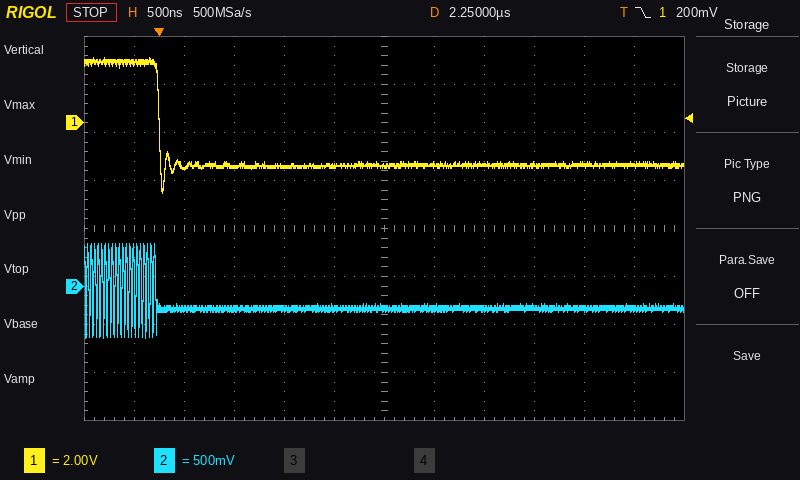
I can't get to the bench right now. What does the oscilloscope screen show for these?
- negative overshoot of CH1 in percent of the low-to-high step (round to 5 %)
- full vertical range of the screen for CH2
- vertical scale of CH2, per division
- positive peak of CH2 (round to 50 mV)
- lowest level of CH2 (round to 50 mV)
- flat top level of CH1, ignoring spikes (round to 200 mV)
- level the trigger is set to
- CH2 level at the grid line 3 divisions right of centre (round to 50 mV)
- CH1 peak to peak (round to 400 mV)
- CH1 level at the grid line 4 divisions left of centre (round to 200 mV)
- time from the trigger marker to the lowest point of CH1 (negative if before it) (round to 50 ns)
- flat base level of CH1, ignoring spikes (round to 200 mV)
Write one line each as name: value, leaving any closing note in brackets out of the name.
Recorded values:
negative overshoot of CH1 in percent of the low-to-high step: 25 %
full vertical range of the screen for CH2: 4 V
vertical scale of CH2, per division: 500 mV
positive peak of CH2: 450 mV
lowest level of CH2: -550 mV
flat top level of CH1, ignoring spikes: 2.6 V
level the trigger is set to: 200 mV
CH2 level at the grid line 3 divisions right of centre: -200 mV
CH1 peak to peak: 5.6 V
CH1 level at the grid line 4 divisions left of centre: -1.8 V
time from the trigger marker to the lowest point of CH1 (negative if before it): +50 ns
flat base level of CH1, ignoring spikes: -1.8 V
